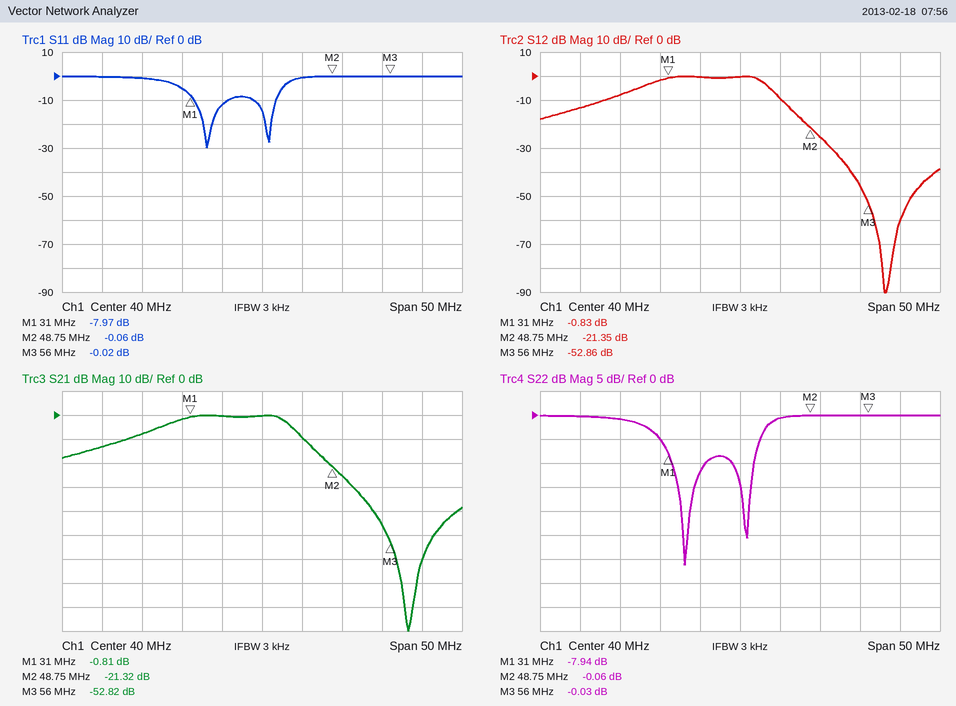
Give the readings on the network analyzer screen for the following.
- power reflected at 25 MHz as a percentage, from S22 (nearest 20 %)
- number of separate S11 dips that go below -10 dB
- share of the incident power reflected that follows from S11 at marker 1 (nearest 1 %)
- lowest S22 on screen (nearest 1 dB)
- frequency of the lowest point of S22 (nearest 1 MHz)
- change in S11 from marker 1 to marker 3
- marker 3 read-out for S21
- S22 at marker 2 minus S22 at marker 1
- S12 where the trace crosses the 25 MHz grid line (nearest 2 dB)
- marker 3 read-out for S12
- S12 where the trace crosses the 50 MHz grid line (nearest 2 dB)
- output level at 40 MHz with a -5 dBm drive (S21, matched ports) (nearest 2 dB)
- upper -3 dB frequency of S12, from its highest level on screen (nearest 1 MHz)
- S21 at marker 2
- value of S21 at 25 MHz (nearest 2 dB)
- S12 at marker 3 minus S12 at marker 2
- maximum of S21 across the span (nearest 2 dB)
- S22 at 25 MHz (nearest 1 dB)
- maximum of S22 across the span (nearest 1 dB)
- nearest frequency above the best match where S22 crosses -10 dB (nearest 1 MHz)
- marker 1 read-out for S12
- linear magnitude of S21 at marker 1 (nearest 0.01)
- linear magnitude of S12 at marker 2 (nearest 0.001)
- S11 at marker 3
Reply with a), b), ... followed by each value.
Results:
a) 80 %
b) 2
c) 16 %
d) -31 dB
e) 33 MHz
f) 7.95 dB
g) -52.82 dB
h) 7.88 dB
i) -8 dB
j) -52.86 dB
k) -26 dB
l) -6 dBm
m) 43 MHz
n) -21.32 dB
o) -8 dB
p) -31.51 dB
q) 0 dB
r) -1 dB
s) 0 dB
t) 36 MHz
u) -0.83 dB
v) 0.91
w) 0.086
x) -0.02 dB
